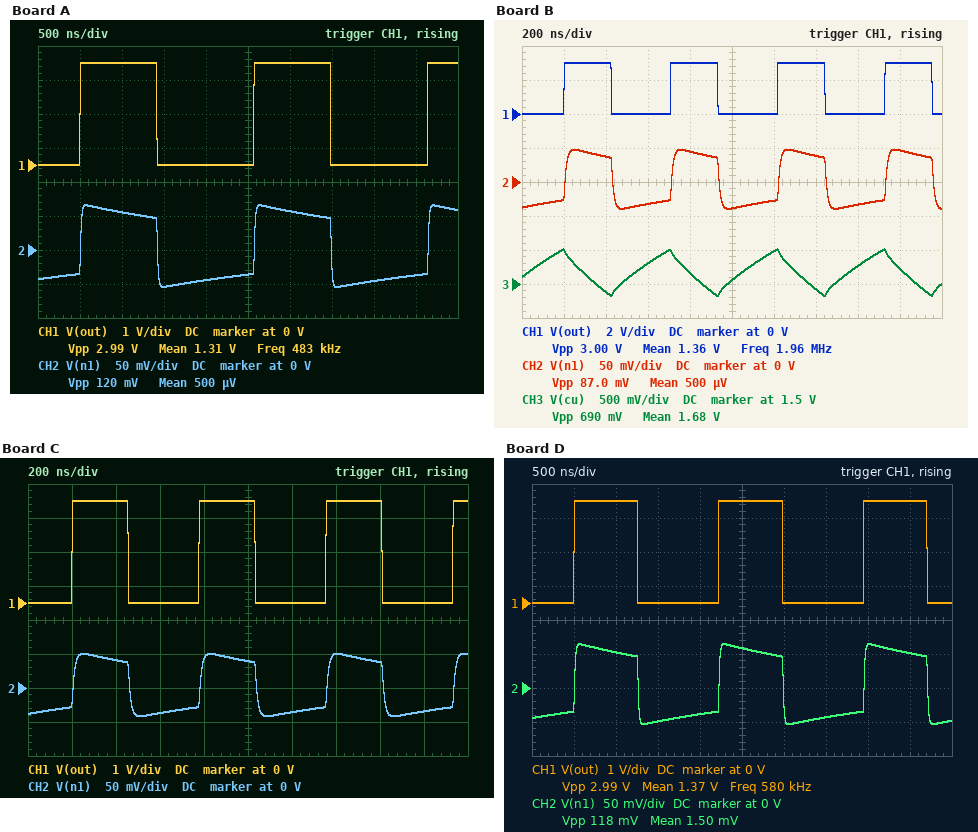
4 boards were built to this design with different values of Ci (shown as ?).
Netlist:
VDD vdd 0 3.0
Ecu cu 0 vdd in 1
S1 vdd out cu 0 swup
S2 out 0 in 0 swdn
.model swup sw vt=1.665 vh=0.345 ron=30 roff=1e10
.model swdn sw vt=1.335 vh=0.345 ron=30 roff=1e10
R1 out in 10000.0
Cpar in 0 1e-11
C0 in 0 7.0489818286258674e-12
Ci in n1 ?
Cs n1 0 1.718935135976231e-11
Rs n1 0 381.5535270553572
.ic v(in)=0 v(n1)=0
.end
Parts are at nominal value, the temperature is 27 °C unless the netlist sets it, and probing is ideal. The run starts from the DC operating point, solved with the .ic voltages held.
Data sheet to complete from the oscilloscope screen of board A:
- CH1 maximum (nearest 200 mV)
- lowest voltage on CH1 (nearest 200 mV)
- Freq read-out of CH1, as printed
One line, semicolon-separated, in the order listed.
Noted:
3.0 V; 0 V; 483 kHz
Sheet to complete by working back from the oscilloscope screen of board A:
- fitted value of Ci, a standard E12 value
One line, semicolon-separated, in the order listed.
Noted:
220 pF
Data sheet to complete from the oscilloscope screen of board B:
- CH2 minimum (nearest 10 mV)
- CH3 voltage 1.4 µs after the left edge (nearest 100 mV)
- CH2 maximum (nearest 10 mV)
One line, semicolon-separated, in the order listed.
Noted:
-40 mV; 1.4 V; 50 mV
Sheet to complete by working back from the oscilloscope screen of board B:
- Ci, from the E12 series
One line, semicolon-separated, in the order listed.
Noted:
39 pF
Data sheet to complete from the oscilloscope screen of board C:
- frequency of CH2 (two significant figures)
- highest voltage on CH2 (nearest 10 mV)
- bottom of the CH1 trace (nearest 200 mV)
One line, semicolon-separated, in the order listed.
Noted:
1.7 MHz; 50 mV; 0 V
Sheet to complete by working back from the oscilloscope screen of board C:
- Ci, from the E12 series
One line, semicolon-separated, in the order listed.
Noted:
47 pF
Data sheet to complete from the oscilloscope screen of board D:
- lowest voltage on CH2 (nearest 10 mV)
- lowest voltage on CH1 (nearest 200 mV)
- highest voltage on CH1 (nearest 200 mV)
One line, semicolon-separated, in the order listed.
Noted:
-50 mV; 0 V; 3.0 V
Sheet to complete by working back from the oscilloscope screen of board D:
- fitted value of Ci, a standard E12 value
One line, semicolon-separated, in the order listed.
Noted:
180 pF
